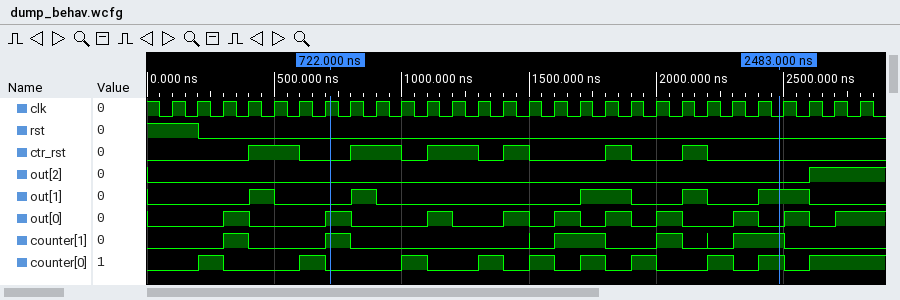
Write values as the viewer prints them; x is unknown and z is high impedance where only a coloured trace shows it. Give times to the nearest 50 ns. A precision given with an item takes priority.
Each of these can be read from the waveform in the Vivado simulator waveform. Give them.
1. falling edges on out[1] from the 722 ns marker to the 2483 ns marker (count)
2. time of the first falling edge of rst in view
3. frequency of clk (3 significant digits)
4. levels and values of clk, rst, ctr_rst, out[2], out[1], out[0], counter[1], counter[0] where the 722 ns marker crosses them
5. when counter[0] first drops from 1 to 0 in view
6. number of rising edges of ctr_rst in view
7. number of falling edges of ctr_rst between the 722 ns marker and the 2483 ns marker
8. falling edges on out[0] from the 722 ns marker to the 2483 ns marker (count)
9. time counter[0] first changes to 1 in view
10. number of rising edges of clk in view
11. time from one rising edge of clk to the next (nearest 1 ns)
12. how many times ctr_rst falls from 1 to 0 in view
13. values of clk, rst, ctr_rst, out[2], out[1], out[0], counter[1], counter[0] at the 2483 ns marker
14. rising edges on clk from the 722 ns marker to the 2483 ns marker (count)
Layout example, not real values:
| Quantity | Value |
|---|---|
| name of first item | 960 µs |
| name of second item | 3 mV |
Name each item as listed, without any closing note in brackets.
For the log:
| Quantity | Value |
|---|---|
| falling edges on out[1] from the 722 ns marker to the 2483 ns marker | 3 |
| time of the first falling edge of rst in view | 200 ns |
| frequency of clk | 10.0 MHz |
| levels and values of clk, rst, ctr_rst, out[2], out[1], out[0], counter[1], counter[0] where the 722 ns marker crosses them | clk=1, rst=0, ctr_rst=0, out[2]=0, out[1]=0, out[0]=1, counter[1]=1, counter[0]=0 |
| when counter[0] first drops from 1 to 0 in view | 300 ns |
| number of rising edges of ctr_rst in view | 6 |
| number of falling edges of ctr_rst between the 722 ns marker and the 2483 ns marker | 5 |
| falling edges on out[0] from the 722 ns marker to the 2483 ns marker | 7 |
| time counter[0] first changes to 1 in view | 200 ns |
| number of rising edges of clk in view | 28 |
| time from one rising edge of clk to the next | 100 ns |
| how many times ctr_rst falls from 1 to 0 in view | 6 |
| values of clk, rst, ctr_rst, out[2], out[1], out[0], counter[1], counter[0] at the 2483 ns marker | clk=0, rst=0, ctr_rst=0, out[2]=0, out[1]=1, out[0]=0, counter[1]=1, counter[0]=1 |
| rising edges on clk from the 722 ns marker to the 2483 ns marker | 17 |
